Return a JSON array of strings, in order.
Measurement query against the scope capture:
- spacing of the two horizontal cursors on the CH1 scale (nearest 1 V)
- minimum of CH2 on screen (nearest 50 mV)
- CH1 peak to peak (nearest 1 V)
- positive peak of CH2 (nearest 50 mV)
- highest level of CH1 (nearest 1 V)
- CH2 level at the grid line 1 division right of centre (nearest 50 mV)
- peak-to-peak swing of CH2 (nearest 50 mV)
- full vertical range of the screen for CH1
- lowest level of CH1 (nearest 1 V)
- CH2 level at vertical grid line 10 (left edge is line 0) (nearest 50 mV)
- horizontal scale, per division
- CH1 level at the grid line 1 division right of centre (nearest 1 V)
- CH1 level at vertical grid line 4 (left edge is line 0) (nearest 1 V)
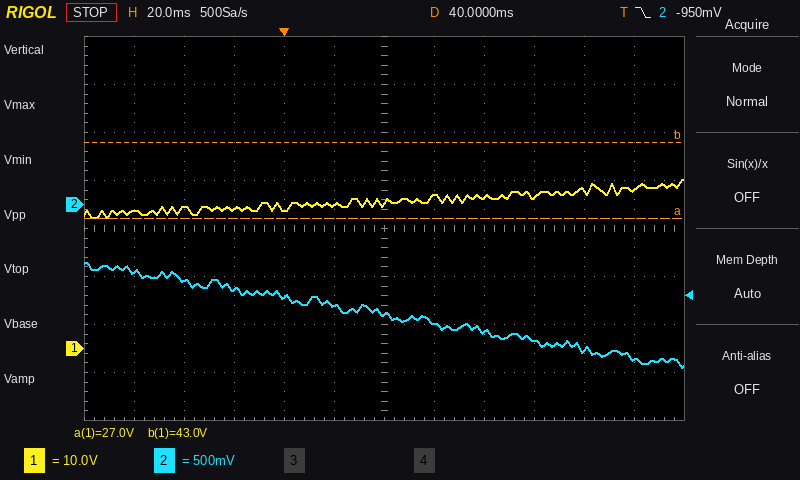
["16 V", "-1.70 V", "8 V", "-600 mV", "35 V", "-1.25 V", "1.10 V", "80 V", "27 V", "-1.50 V", "20 ms", "32 V", "29 V"]
